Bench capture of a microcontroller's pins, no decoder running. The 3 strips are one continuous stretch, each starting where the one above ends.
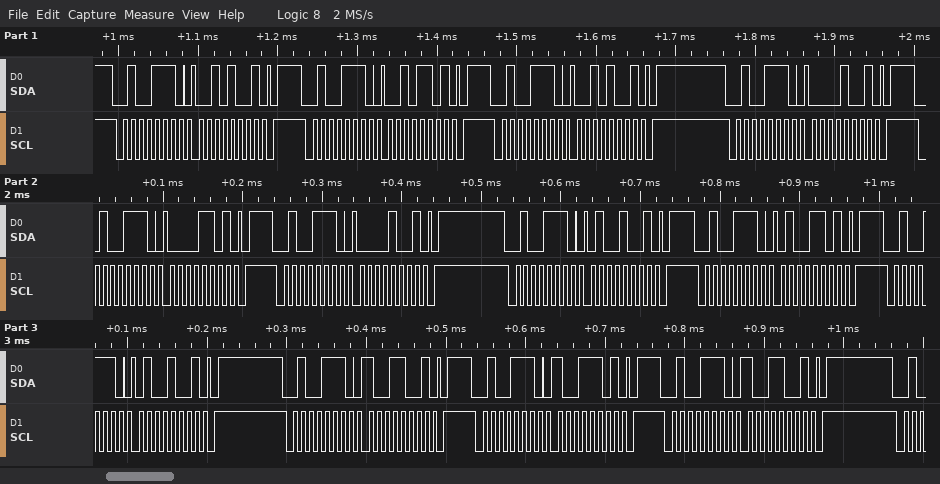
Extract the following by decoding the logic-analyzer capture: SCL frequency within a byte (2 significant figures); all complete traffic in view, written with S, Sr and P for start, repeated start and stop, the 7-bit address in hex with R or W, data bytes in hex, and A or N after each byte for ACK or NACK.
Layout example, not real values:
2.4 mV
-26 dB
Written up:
100 kHz
S 27W A 29 A P S 27W A 2D A P S 27W A 29 A P S 27W A 09 A P S 27W A 0D A P S 27W A 09 A P S 27W A 49 A P S 27W A 4D A P S 27W A 49 A P S 27W A 99 A P S 27W A 9D A P S 27W A 99 A P
